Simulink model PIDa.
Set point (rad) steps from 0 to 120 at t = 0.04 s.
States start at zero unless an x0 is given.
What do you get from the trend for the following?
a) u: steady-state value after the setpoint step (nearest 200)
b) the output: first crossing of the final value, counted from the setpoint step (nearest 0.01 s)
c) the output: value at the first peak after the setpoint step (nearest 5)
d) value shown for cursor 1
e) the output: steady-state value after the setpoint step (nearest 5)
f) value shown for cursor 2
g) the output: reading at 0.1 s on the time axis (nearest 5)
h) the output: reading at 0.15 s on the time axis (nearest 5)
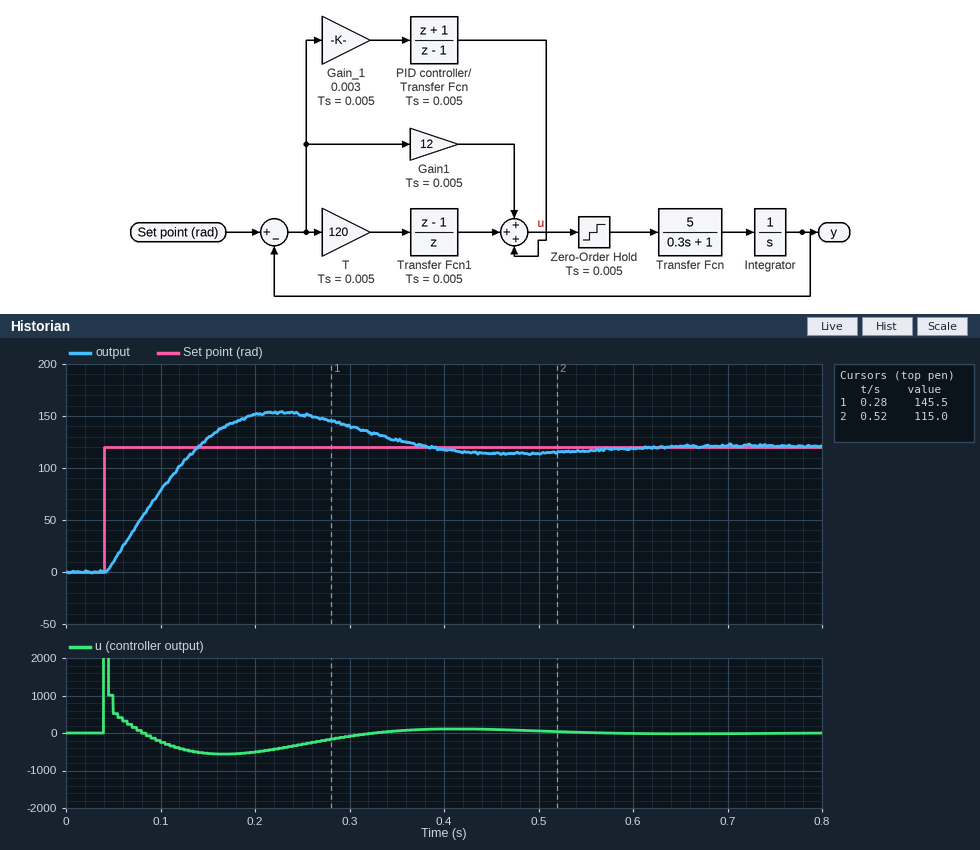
0
0.10 s
155
145.5
120
115.0
80
130
